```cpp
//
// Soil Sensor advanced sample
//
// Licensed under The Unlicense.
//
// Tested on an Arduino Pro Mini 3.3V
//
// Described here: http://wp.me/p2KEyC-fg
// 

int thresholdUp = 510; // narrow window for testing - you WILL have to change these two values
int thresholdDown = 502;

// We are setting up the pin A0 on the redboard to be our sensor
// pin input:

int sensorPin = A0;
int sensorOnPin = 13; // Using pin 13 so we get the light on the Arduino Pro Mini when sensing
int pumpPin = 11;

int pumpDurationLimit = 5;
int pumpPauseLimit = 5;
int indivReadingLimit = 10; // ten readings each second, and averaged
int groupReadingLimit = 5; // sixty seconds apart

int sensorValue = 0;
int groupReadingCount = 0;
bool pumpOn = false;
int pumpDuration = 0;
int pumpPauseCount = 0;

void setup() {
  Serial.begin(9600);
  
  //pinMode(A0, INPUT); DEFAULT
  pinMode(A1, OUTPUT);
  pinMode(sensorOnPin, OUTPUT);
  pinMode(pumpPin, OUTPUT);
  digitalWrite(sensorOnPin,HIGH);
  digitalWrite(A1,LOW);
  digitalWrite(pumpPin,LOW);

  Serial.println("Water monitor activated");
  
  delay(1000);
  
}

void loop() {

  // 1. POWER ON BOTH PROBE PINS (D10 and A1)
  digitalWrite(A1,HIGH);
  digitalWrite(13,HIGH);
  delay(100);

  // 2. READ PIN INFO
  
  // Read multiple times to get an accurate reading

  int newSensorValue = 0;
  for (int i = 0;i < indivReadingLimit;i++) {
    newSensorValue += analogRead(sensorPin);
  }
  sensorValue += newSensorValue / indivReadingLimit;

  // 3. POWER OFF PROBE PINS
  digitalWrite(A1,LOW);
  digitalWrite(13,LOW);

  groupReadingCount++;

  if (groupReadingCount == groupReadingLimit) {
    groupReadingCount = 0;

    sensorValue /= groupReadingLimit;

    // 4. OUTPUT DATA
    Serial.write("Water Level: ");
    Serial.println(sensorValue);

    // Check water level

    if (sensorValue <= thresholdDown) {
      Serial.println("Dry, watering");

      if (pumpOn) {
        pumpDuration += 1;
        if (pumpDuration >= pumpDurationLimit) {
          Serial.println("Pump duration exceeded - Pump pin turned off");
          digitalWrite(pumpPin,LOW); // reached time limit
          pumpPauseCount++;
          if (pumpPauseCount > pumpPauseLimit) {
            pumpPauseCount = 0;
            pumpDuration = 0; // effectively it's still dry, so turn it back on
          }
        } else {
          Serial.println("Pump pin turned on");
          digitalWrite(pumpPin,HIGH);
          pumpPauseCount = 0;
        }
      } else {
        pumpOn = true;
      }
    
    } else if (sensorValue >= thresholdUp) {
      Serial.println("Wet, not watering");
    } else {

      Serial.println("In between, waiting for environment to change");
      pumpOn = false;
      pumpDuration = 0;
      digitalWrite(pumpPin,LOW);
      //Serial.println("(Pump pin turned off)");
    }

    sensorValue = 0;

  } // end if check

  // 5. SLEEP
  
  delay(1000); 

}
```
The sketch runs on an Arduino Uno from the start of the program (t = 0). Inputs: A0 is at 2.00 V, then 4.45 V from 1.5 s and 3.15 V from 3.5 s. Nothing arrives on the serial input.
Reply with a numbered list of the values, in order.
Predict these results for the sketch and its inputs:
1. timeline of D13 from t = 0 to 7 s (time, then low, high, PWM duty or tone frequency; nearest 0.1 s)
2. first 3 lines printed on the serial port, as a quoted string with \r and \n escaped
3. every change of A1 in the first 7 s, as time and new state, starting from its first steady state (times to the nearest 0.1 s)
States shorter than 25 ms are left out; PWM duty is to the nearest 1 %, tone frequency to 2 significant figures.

1. 0 s high; 1.1 s low; 2.1 s high; 2.2 s low; 3.2 s high; 3.3 s low; 4.3 s high; 4.4 s low; 5.4 s high; 5.5 s low; 6.5 s high; 6.6 s low
2. "Water monitor activated\r\nWater Level: 704\r\nWet, not watering\r\n"
3. 0 s low; 1 s high; 1.1 s low; 2.1 s high; 2.2 s low; 3.2 s high; 3.3 s low; 4.3 s high; 4.4 s low; 5.4 s high; 5.5 s low; 6.5 s high; 6.6 s low
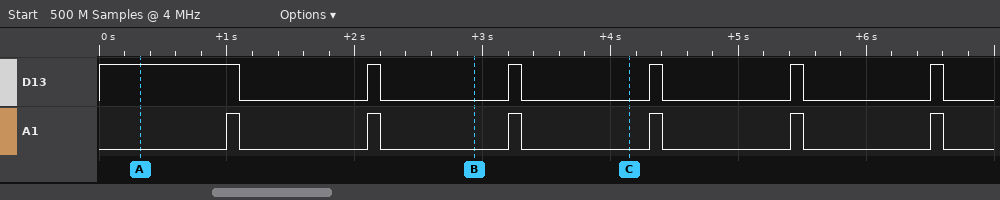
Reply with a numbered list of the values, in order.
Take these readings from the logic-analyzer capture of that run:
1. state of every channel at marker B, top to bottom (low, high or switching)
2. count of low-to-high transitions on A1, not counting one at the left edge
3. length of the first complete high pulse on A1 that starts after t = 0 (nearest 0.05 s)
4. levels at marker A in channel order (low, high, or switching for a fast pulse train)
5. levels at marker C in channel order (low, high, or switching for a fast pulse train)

1. D13 low, A1 low
2. 6
3. 0.10 s
4. D13 high, A1 low
5. D13 low, A1 low
